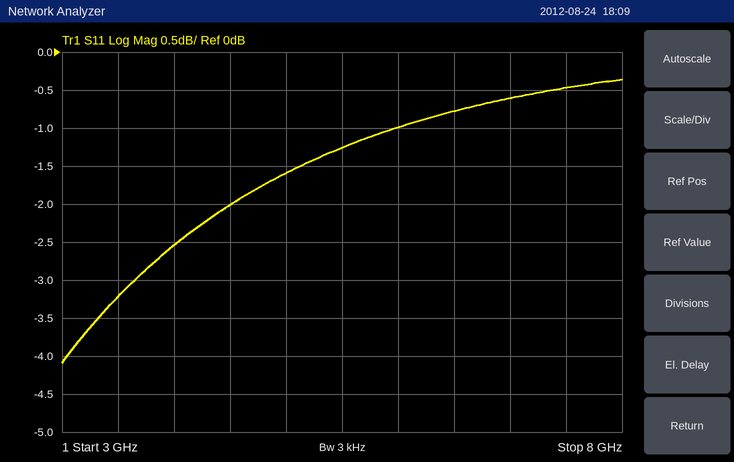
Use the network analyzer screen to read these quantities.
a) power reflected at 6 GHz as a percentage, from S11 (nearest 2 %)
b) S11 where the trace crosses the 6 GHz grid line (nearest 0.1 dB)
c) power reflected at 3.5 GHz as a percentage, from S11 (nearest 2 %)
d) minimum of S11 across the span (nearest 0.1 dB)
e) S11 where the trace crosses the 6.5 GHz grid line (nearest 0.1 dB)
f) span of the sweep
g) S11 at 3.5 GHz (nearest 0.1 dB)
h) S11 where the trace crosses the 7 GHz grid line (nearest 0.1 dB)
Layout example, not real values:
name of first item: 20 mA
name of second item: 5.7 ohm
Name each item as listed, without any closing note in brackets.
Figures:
power reflected at 6 GHz as a percentage, from S11: 80 %
S11 where the trace crosses the 6 GHz grid line: -1.0 dB
power reflected at 3.5 GHz as a percentage, from S11: 48 %
minimum of S11 across the span: -4.1 dB
S11 where the trace crosses the 6.5 GHz grid line: -0.8 dB
span of the sweep: 5 GHz
S11 at 3.5 GHz: -3.2 dB
S11 where the trace crosses the 7 GHz grid line: -0.6 dB
